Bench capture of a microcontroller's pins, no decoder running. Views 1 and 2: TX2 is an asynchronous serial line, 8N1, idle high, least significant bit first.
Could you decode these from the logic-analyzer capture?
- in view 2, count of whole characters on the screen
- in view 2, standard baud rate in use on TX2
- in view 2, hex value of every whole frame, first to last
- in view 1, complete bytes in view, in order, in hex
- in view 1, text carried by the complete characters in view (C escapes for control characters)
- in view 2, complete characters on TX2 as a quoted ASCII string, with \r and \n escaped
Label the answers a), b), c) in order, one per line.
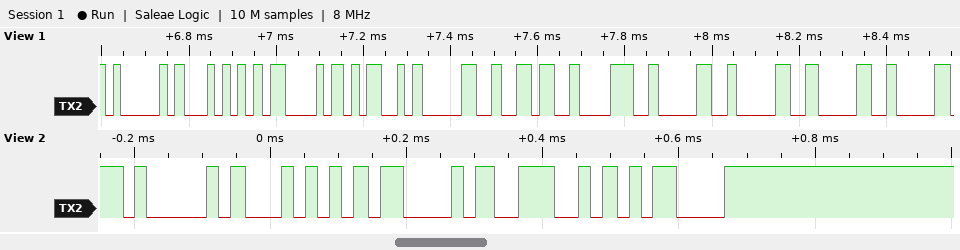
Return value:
a) 5
b) 57600 baud
c) 41 54 43 4E 0D
d) 0x41 0x54 0x43 0x4D 0x30 0x36 0x38 0x30 0x30 0x30
e) "ATCM068000"
f) "ATCN\r"
